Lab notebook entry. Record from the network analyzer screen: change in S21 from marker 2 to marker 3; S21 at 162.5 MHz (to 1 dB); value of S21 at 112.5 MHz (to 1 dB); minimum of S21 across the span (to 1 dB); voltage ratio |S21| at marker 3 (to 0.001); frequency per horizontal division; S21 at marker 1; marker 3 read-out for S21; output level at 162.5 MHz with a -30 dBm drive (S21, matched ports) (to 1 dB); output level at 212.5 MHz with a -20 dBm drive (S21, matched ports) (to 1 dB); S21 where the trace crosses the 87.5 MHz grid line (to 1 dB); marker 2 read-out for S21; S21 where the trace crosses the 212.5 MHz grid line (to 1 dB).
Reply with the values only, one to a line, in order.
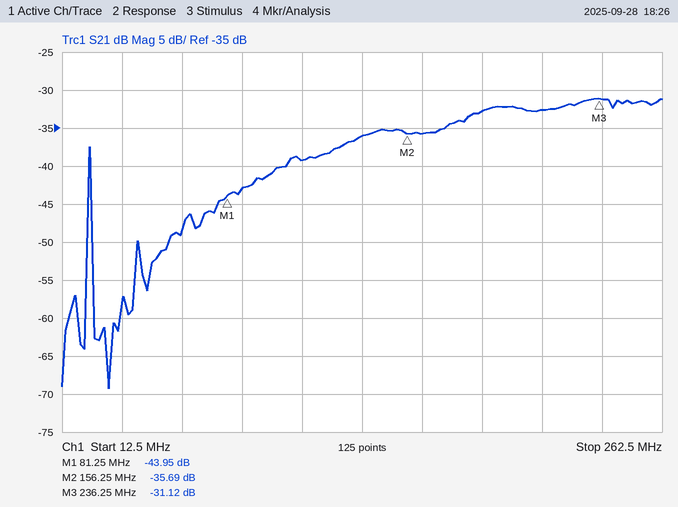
4.57 dB
-36 dB
-39 dB
-69 dB
0.028
25 MHz
-43.95 dB
-31.12 dB
-66 dBm
-53 dBm
-43 dB
-35.69 dB
-33 dB
